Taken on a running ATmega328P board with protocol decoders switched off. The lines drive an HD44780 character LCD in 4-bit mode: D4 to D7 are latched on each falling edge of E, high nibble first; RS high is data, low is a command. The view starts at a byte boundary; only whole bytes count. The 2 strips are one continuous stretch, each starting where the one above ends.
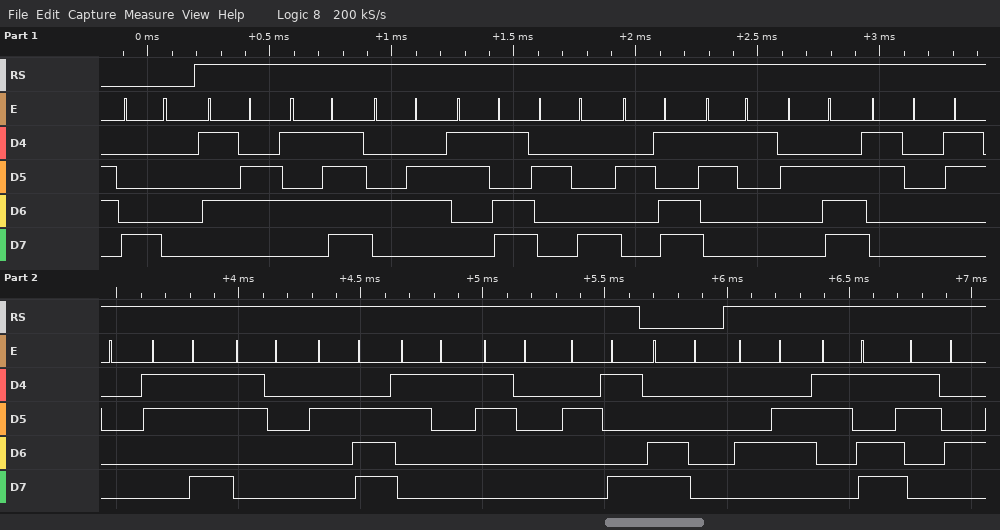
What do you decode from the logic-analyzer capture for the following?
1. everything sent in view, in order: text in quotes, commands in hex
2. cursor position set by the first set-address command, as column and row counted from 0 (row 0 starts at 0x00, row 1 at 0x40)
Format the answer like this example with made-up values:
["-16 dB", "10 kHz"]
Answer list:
["0x80 \"V_F=(-1.00;0.10)\" 0xC0 \"F=4\"", "column 0, row 0"]
